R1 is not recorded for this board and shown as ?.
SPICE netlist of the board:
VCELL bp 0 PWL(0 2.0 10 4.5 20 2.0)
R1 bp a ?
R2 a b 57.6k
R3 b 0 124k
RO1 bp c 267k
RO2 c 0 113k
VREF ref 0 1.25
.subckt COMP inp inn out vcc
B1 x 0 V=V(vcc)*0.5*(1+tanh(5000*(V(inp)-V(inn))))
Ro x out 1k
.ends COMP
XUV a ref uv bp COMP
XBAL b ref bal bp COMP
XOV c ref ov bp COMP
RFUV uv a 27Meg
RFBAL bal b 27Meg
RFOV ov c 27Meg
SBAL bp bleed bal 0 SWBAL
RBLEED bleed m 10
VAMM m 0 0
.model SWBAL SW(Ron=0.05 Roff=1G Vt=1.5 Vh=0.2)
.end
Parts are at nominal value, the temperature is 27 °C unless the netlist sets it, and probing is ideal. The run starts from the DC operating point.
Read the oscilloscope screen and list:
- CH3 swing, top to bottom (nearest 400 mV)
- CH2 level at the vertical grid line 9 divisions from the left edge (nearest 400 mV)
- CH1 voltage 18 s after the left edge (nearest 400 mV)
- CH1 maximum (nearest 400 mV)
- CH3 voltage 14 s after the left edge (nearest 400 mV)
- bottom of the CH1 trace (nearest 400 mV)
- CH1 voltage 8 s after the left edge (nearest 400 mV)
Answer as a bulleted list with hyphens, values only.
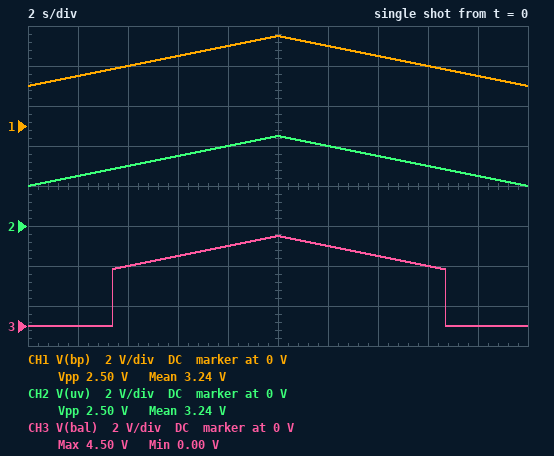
- 4.4 V
- 2.4 V
- 2.4 V
- 4.4 V
- 3.6 V
- 2.0 V
- 4.0 V
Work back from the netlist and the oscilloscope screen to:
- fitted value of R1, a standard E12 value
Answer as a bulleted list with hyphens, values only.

- 100 kΩ
